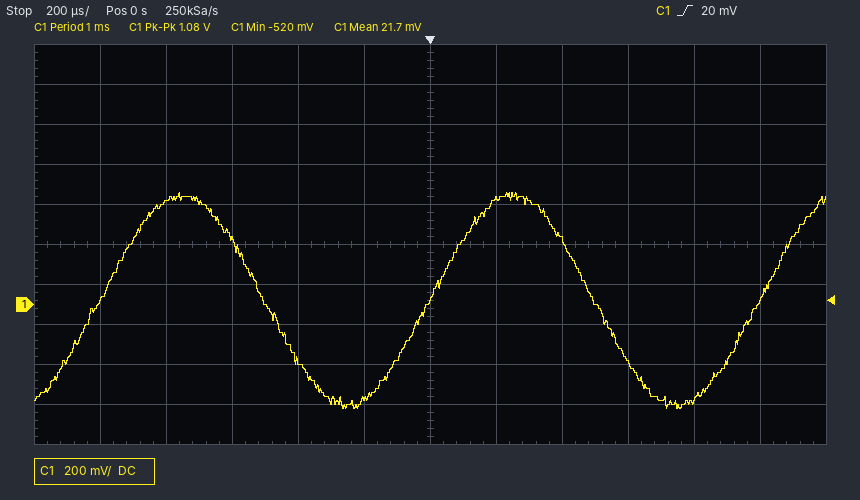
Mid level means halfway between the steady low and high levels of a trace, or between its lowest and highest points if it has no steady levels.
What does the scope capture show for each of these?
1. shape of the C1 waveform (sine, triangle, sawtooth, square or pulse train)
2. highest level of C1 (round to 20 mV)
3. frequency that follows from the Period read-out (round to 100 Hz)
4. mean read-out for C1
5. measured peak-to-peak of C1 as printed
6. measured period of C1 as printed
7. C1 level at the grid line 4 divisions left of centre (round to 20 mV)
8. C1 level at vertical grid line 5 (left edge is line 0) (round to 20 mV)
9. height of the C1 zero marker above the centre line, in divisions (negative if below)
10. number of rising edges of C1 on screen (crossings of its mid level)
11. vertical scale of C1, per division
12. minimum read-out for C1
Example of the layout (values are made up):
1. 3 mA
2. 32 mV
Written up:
1. sine
2. 560 mV
3. 1.0 kHz
4. 21.7 mV
5. 1.08 V
6. 1 ms
7. 520 mV
8. -480 mV
9. -1.5 div
10. 3
11. 200 mV
12. -520 mV
